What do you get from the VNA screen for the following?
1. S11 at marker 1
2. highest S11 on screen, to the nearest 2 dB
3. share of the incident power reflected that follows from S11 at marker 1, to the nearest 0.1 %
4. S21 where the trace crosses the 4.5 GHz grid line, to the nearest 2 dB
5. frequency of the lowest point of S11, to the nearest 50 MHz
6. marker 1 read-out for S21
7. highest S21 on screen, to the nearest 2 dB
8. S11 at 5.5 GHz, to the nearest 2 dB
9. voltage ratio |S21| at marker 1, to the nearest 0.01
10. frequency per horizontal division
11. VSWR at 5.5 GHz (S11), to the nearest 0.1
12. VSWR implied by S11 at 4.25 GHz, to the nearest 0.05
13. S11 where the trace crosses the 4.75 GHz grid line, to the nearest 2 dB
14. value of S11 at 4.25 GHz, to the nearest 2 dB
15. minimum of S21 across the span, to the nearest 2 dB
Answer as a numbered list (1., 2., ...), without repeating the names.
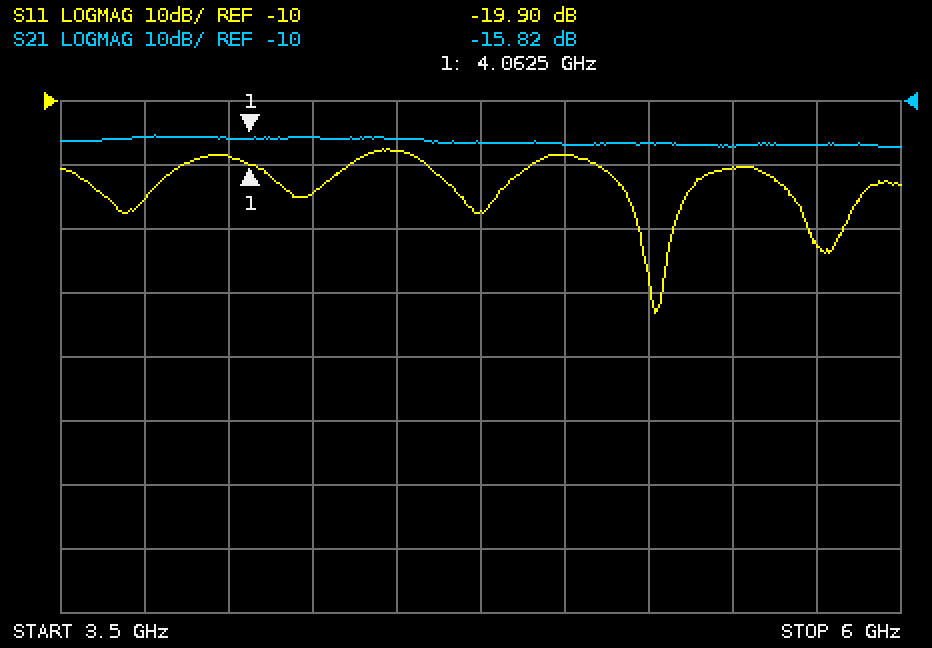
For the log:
1. -19.90 dB
2. -18 dB
3. 1.0 %
4. -16 dB
5. 5.25 GHz
6. -15.82 dB
7. -16 dB
8. -20 dB
9. 0.16
10. 250 MHz
11. 1.2
12. 1.15
13. -28 dB
14. -24 dB
15. -18 dB
